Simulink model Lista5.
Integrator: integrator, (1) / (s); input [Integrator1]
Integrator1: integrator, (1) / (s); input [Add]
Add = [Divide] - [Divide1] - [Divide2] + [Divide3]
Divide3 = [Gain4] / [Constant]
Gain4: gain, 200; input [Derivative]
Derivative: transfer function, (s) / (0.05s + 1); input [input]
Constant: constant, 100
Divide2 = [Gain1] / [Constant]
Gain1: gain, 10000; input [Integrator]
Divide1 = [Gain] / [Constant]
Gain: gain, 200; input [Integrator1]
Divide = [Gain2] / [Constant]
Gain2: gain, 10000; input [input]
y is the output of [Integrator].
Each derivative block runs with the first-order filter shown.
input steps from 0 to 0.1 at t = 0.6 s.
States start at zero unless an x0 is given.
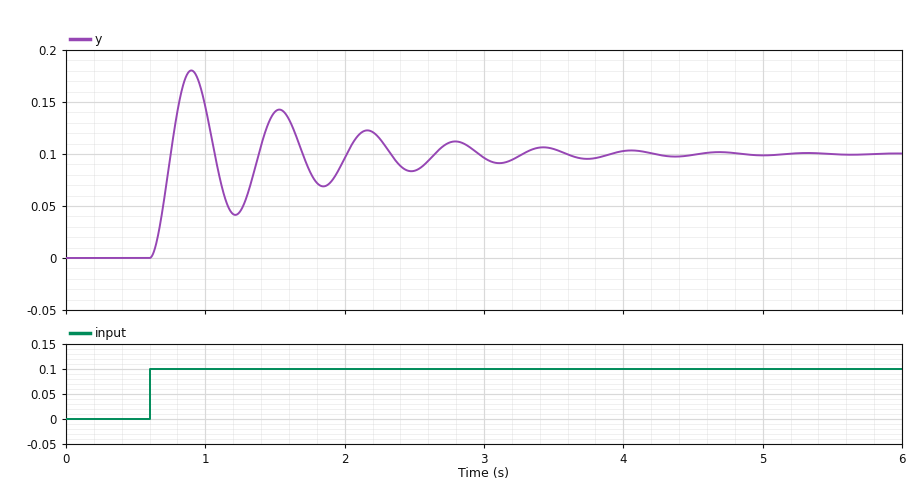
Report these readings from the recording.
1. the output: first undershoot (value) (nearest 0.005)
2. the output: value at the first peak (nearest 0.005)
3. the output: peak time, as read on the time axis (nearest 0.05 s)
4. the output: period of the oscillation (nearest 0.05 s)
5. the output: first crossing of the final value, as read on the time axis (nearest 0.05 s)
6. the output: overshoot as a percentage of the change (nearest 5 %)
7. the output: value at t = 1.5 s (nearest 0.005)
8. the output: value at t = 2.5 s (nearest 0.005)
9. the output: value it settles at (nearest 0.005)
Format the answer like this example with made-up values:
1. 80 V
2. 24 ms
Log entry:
1. 0.040
2. 0.180
3. 0.90 s
4. 0.65 s
5. 0.75 s
6. 80 %
7. 0.140
8. 0.085
9. 0.100
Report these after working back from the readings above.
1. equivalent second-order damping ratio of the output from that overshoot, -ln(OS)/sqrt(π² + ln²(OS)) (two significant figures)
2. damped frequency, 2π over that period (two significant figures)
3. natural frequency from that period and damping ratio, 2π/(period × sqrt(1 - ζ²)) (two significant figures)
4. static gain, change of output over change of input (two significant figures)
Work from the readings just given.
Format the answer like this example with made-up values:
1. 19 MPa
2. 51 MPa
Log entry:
1. 0.071
2. 9.7 rad/s
3. 9.7 rad/s
4. 1.0
